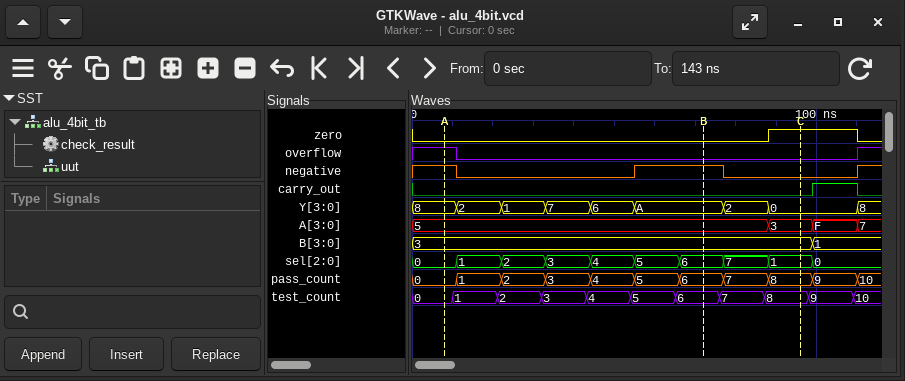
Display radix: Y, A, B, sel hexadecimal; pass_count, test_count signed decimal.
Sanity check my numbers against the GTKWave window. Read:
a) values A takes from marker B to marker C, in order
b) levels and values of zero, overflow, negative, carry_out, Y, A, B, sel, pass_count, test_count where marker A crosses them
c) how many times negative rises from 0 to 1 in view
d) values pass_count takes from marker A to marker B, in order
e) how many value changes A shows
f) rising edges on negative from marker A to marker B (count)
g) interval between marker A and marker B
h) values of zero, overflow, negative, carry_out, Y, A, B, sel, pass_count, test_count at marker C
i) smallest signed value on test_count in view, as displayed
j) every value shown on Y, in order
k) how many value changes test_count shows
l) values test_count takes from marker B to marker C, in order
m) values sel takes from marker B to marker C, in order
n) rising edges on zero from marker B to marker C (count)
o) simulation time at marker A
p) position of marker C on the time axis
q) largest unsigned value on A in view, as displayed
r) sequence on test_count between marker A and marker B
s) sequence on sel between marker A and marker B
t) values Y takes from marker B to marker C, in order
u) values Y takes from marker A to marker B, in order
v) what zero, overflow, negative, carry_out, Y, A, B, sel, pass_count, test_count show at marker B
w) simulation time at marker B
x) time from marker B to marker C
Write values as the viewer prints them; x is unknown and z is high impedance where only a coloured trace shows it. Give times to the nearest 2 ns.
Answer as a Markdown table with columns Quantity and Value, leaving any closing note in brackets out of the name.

| Quantity | Value |
|---|---|
| values A takes from marker B to marker C, in order | 5, 3 |
| levels and values of zero, overflow, negative, carry_out, Y, A, B, sel, pass_count, test_count where marker A crosses them | zero=0, overflow=1, negative=1, carry_out=0, Y=8, A=5, B=3, sel=0, pass_count=0, test_count=0 |
| how many times negative rises from 0 to 1 in view | 2 |
| values pass_count takes from marker A to marker B, in order | 0, 1, 2, 3, 4, 5, 6 |
| how many value changes A shows | 3 |
| rising edges on negative from marker A to marker B | 1 |
| interval between marker A and marker B | 64 ns |
| values of zero, overflow, negative, carry_out, Y, A, B, sel, pass_count, test_count at marker C | zero=1, overflow=0, negative=0, carry_out=0, Y=0, A=3, B=3, sel=1, pass_count=8, test_count=8 |
| smallest signed value on test_count in view, as displayed | 0 |
| every value shown on Y, in order | 8, 2, 1, 7, 6, A, 2, 0, 8 |
| how many value changes test_count shows | 10 |
| values test_count takes from marker B to marker C, in order | 6, 7, 8 |
| values sel takes from marker B to marker C, in order | 6, 7, 1 |
| rising edges on zero from marker B to marker C | 1 |
| simulation time at marker A | 8 ns |
| position of marker C on the time axis | 96 ns |
| largest unsigned value on A in view, as displayed | F |
| sequence on test_count between marker A and marker B | 0, 1, 2, 3, 4, 5, 6 |
| sequence on sel between marker A and marker B | 0, 1, 2, 3, 4, 5, 6 |
| values Y takes from marker B to marker C, in order | A, 2, 0 |
| values Y takes from marker A to marker B, in order | 8, 2, 1, 7, 6, A |
| what zero, overflow, negative, carry_out, Y, A, B, sel, pass_count, test_count show at marker B | zero=0, overflow=0, negative=1, carry_out=0, Y=A, A=5, B=3, sel=6, pass_count=6, test_count=6 |
| simulation time at marker B | 72 ns |
| time from marker B to marker C | 24 ns |
